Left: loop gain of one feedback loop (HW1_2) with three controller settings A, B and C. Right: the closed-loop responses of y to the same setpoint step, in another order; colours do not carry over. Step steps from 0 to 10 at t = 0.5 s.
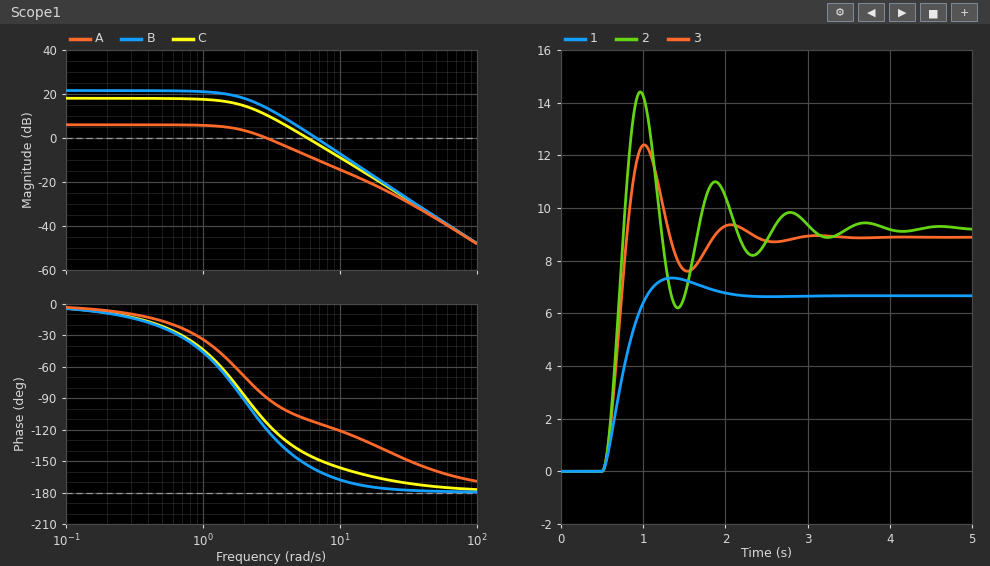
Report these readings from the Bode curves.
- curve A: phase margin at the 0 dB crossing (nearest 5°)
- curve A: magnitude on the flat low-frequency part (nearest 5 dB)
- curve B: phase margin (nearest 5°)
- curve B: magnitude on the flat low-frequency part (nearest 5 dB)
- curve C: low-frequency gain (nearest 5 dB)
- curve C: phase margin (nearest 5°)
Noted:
90°
5 dB
20°
20 dB
20 dB
35°
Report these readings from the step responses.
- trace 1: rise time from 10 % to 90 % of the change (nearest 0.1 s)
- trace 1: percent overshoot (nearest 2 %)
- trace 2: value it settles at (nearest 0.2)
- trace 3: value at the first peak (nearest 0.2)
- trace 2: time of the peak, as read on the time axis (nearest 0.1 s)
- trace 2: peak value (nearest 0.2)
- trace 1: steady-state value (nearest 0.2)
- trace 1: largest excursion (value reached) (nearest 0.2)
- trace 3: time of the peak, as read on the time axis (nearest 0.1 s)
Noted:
0.4 s
10 %
9.2
12.4
1.0 s
14.4
6.6
7.4
1.0 s
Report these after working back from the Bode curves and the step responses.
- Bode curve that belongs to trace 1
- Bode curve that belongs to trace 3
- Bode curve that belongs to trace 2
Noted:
A
C
B
